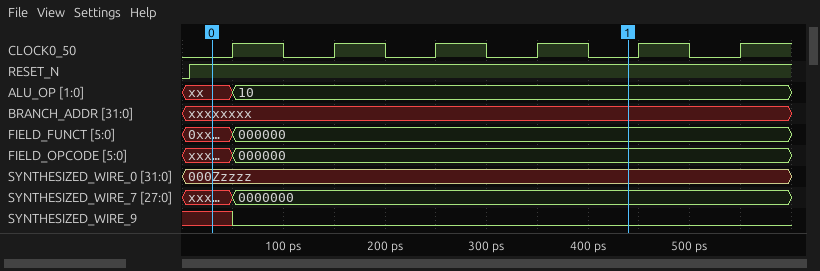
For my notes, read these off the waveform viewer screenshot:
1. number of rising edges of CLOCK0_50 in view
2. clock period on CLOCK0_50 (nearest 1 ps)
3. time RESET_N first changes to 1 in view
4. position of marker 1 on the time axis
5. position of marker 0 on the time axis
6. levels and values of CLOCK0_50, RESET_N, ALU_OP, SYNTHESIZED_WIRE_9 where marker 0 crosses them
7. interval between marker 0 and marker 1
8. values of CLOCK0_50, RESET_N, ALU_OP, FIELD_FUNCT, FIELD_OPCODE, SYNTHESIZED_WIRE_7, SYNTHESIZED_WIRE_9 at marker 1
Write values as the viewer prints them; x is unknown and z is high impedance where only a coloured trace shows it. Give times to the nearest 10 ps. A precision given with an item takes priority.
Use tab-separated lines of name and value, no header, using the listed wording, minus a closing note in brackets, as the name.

number of rising edges of CLOCK0_50 in view	6
clock period on CLOCK0_50	100 ps
time RESET_N first changes to 1 in view	10 ps
position of marker 1 on the time axis	440 ps
position of marker 0 on the time axis	30 ps
levels and values of CLOCK0_50, RESET_N, ALU_OP, SYNTHESIZED_WIRE_9 where marker 0 crosses them	CLOCK0_50=0, RESET_N=1, ALU_OP=xx, SYNTHESIZED_WIRE_9=x
interval between marker 0 and marker 1	410 ps
values of CLOCK0_50, RESET_N, ALU_OP, FIELD_FUNCT, FIELD_OPCODE, SYNTHESIZED_WIRE_7, SYNTHESIZED_WIRE_9 at marker 1	CLOCK0_50=0, RESET_N=1, ALU_OP=10, FIELD_FUNCT=000000, FIELD_OPCODE=000000, SYNTHESIZED_WIRE_7=0000000, SYNTHESIZED_WIRE_9=0
